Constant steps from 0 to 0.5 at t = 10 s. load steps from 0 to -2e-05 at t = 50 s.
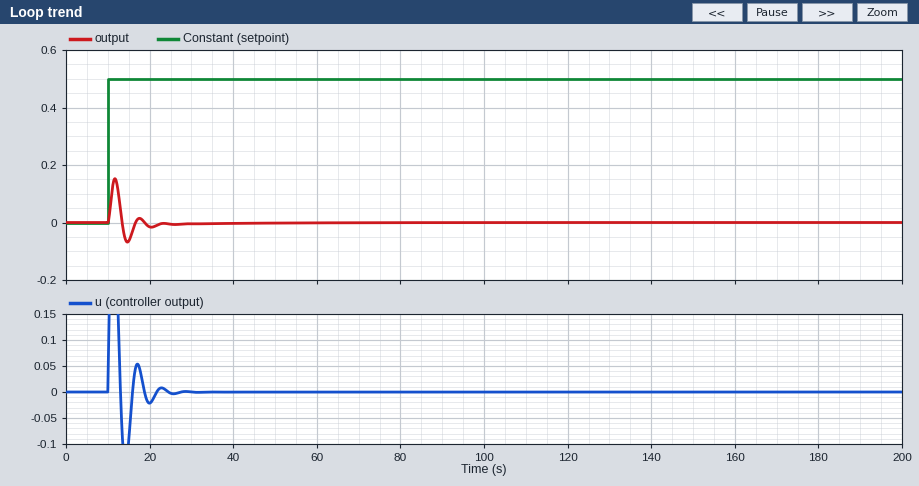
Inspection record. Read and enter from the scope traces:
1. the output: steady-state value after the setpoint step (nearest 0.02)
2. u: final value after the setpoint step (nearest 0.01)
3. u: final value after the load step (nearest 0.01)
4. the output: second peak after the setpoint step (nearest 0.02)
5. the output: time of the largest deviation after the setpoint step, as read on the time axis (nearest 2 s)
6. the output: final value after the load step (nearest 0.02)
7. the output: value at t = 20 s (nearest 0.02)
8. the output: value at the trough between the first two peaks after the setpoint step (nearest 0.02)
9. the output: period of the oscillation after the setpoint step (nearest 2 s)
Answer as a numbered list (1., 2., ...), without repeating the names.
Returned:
1. 0.00
2. 0.00
3. 0.00
4. 0.02
5. 12 s
6. 0.00
7. -0.02
8. -0.06
9. 6 s
